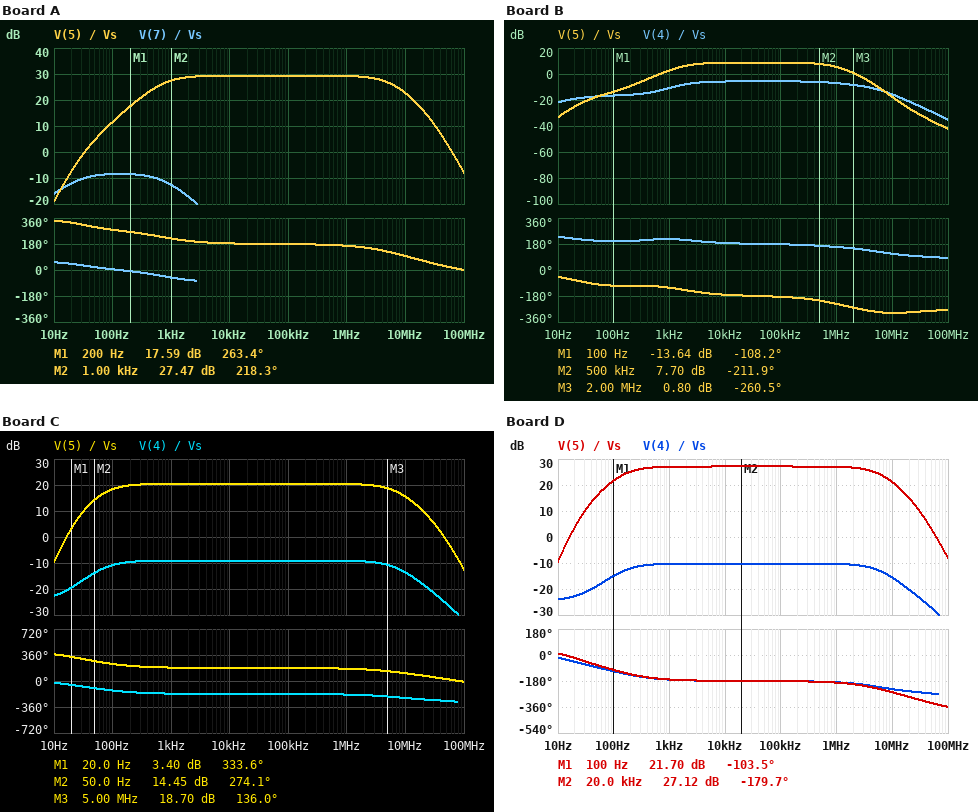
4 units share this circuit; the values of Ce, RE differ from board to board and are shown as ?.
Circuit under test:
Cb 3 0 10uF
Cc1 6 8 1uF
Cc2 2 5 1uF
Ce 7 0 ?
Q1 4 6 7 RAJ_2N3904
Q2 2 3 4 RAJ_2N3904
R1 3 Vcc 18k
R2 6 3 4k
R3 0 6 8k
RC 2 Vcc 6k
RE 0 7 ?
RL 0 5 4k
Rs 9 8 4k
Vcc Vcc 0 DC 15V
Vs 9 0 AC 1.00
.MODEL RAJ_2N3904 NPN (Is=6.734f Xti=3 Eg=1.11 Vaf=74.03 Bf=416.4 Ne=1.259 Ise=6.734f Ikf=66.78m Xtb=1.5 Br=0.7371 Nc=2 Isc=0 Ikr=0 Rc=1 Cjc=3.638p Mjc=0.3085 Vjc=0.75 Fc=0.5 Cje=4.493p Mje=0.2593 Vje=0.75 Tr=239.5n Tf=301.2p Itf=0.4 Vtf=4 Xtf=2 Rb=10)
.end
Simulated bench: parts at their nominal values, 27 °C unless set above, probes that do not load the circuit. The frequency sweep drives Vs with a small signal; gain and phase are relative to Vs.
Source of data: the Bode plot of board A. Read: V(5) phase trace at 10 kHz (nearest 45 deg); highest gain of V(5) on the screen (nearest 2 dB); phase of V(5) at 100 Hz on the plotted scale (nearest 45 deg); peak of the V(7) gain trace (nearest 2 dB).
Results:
180 deg
30 dB
270 deg
-8 dB
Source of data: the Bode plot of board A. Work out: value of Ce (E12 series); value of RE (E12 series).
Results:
6.8 µF
2.7 kΩ
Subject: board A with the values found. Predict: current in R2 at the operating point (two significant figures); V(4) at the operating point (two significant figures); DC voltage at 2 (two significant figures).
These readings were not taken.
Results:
500 µA
5.2 V
7.9 V
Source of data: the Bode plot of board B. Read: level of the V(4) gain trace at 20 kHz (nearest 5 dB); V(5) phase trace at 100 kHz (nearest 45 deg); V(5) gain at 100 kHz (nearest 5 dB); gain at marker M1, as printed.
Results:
-5 dB
-180 deg
10 dB
-13.64 dB
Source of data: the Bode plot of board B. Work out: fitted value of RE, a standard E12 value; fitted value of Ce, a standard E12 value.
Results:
1.2 kΩ
4.7 µF
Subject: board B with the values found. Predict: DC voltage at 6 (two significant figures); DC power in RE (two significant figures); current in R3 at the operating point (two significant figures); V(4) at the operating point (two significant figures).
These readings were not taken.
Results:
3.1 V
4.8 mW
390 µA
4.0 V
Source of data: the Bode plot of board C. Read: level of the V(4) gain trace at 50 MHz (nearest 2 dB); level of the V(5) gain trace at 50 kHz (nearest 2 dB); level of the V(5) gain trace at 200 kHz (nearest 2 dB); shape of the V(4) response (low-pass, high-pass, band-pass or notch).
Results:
-26 dB
20 dB
20 dB
band-pass
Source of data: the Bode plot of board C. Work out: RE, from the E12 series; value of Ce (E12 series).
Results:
10 kΩ
27 µF
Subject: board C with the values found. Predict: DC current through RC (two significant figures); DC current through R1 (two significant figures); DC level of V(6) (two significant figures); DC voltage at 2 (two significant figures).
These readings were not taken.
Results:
330 µA
500 µA
4.0 V
13 V
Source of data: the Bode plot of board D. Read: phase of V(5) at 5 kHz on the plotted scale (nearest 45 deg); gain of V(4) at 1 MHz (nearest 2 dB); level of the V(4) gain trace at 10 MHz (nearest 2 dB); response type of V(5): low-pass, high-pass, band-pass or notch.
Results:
-180 deg
-10 dB
-16 dB
band-pass
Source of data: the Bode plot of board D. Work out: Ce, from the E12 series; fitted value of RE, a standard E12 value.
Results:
27 µF
3.9 kΩ
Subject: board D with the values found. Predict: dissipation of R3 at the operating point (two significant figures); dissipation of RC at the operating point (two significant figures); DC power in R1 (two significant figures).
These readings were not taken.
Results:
1.9 mW
4.1 mW
4.6 mW
